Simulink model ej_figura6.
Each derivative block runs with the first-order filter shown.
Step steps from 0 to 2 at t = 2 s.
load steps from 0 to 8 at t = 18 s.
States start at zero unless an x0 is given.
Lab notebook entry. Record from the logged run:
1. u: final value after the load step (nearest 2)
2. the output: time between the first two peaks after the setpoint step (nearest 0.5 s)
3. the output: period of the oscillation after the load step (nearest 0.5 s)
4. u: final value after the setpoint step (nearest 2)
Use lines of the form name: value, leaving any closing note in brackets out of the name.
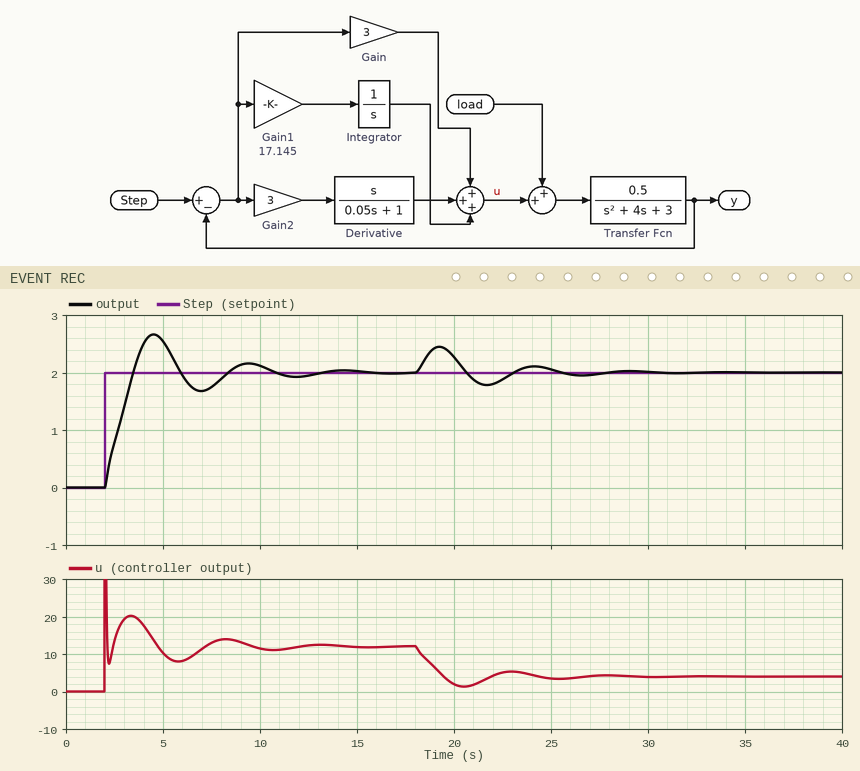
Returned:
u: final value after the load step: 4
the output: time between the first two peaks after the setpoint step: 5.0 s
the output: period of the oscillation after the load step: 5.0 s
u: final value after the setpoint step: 12
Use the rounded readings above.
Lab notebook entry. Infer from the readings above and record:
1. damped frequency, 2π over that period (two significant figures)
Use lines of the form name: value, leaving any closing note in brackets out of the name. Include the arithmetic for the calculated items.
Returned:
damped frequency, 2π over that period: 2π / 5 = 1.3 rad/s
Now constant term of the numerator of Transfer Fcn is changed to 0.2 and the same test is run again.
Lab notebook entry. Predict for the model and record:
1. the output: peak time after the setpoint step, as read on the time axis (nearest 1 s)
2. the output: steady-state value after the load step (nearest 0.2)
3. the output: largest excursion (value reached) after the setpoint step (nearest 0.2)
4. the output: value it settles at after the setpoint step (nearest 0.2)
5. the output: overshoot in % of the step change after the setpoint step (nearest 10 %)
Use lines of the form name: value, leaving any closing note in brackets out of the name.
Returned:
the output: peak time after the setpoint step, as read on the time axis: 6 s
the output: steady-state value after the load step: 2.0
the output: largest excursion (value reached) after the setpoint step: 2.4
the output: value it settles at after the setpoint step: 2.0
the output: overshoot in % of the step change after the setpoint step: 20 %
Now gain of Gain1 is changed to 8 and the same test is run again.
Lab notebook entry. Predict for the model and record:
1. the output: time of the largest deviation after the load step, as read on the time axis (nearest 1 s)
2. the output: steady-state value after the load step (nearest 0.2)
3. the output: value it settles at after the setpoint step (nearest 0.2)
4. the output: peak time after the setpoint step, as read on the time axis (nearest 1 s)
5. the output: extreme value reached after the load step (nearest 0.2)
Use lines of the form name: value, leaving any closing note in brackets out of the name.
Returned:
the output: time of the largest deviation after the load step, as read on the time axis: 20 s
the output: steady-state value after the load step: 2.0
the output: value it settles at after the setpoint step: 2.0
the output: peak time after the setpoint step, as read on the time axis: 6 s
the output: extreme value reached after the load step: 2.6
